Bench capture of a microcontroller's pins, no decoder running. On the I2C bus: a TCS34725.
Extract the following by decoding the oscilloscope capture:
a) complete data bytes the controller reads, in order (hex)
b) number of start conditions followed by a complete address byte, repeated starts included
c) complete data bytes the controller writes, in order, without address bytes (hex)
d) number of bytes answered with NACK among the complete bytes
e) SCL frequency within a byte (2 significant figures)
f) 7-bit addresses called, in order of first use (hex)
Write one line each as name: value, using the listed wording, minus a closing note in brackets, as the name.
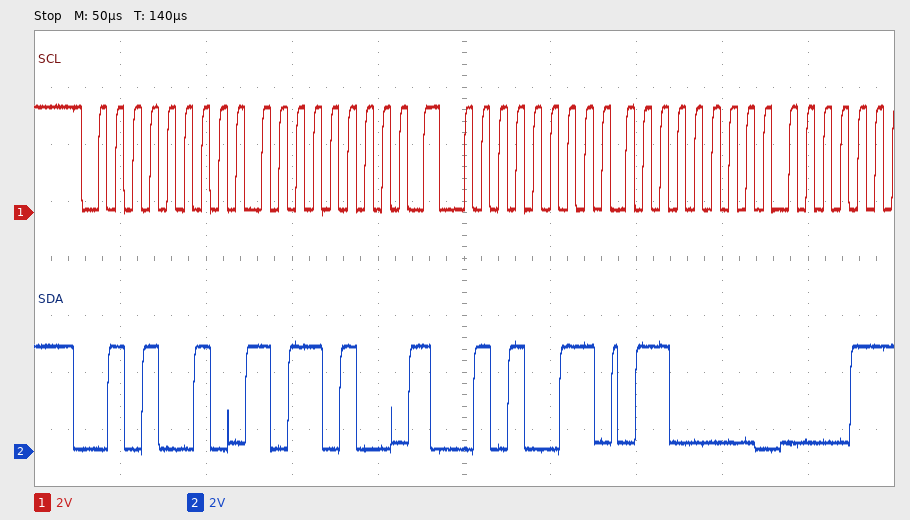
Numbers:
complete data bytes the controller reads, in order: 60
number of start conditions followed by a complete address byte, repeated starts included: 2
complete data bytes the controller writes, in order, without address bytes: B4
number of bytes answered with NACK among the complete bytes: 0
SCL frequency within a byte: 100 kHz
7-bit addresses called, in order of first use: 0x29
